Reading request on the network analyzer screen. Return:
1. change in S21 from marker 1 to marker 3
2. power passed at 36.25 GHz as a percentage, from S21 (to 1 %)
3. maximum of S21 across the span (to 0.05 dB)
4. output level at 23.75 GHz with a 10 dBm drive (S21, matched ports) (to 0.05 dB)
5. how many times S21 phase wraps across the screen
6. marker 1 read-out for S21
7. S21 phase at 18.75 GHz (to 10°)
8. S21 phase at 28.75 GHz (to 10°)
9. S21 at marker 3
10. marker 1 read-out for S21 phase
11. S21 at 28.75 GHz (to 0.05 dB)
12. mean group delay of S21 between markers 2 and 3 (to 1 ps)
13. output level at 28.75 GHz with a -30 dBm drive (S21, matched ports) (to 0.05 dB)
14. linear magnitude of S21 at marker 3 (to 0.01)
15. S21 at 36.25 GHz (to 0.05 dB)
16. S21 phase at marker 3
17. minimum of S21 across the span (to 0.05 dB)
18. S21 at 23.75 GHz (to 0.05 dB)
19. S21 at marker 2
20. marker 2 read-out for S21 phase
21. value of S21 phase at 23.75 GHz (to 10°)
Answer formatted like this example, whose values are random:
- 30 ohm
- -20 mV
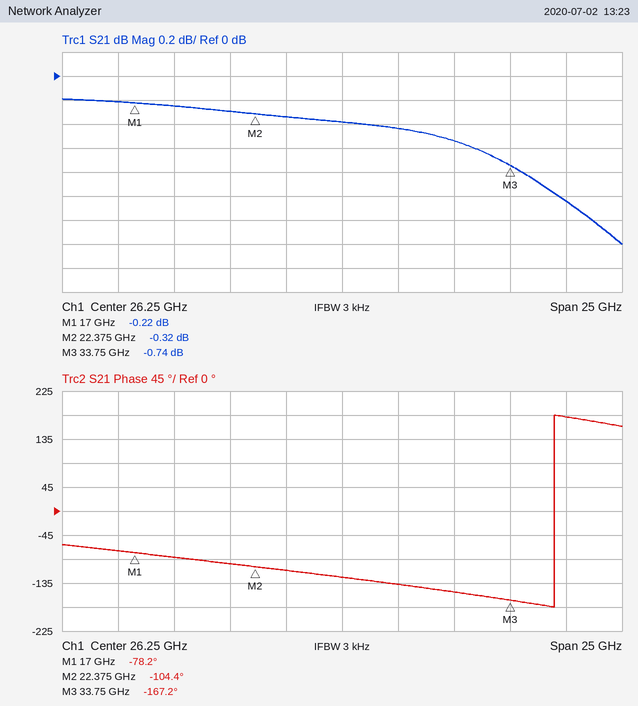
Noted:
- -0.52 dB
- 79 %
- -0.20 dB
- 9.65 dBm
- 1
- -0.22 dB
- -90°
- -140°
- -0.74 dB
- -78.2°
- -0.45 dB
- 15 ps
- -30.45 dBm
- 0.92
- -1.05 dB
- -167.2°
- -1.40 dB
- -0.35 dB
- -0.32 dB
- -104.4°
- -110°
